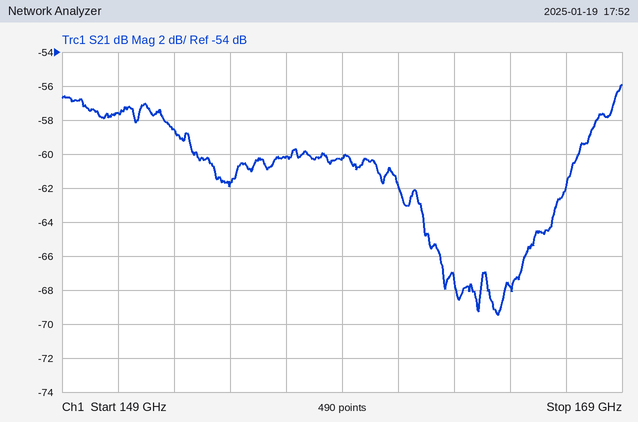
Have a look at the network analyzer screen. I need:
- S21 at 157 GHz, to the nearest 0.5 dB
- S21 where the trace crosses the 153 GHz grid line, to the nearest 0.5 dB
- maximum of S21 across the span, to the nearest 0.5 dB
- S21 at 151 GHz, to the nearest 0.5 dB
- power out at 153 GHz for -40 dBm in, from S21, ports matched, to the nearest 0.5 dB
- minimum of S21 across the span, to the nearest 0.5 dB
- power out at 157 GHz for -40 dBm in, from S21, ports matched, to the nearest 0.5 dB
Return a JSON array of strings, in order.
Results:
["-60.0 dB", "-58.5 dB", "-56.0 dB", "-57.5 dB", "-98.5 dBm", "-69.5 dB", "-100.0 dBm"]
